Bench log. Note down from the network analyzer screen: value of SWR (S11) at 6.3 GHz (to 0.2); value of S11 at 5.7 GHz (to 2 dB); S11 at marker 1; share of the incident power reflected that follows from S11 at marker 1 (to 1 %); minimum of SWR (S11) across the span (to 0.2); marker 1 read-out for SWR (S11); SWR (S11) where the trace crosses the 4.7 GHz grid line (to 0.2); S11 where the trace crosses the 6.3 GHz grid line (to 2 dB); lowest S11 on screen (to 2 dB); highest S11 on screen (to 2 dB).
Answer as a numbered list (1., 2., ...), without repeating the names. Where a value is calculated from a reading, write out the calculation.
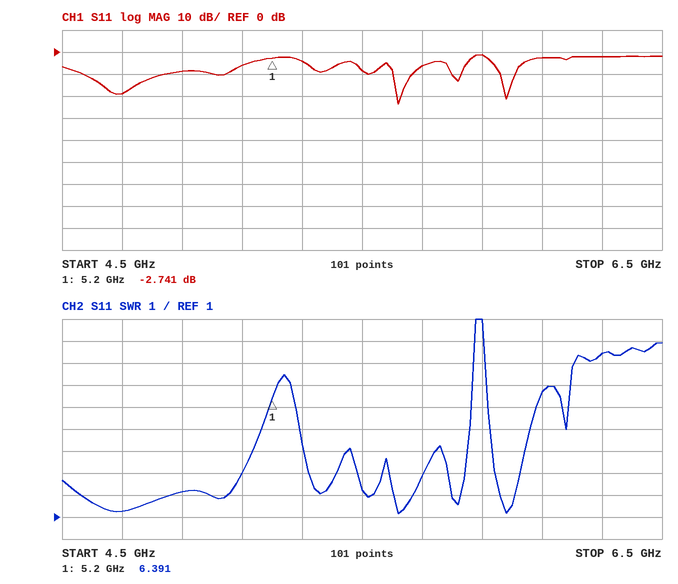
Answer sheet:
1. 8.4
2. -6 dB
3. -2.741 dB
4. 10^(-2.741/10) ≈ 53 %
5. 1.2
6. 6.391
7. 1.2
8. -2 dB
9. -24 dB
10. -2 dB
